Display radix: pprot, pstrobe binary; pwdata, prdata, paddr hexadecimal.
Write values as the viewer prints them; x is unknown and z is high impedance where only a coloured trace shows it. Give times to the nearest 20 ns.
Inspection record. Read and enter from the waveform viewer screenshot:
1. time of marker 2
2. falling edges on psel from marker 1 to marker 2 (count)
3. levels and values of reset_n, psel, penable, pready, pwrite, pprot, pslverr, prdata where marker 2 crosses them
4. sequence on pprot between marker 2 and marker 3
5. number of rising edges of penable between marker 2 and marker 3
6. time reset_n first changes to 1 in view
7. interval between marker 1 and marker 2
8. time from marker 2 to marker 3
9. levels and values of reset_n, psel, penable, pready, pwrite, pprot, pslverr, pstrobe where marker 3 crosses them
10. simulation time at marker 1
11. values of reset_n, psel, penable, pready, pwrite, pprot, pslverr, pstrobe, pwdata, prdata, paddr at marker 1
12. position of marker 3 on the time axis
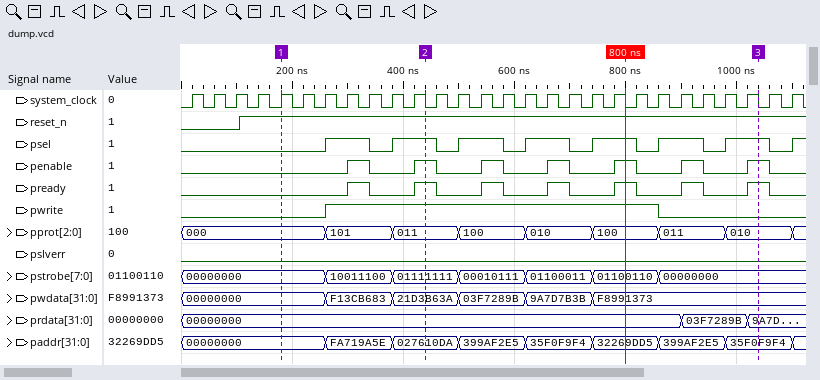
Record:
440 ns
1
reset_n=1, psel=1, penable=1, pready=1, pwrite=1, pprot=011, pslverr=0, prdata=00000000
011, 100, 010, 100, 011, 010
5
100 ns
260 ns
600 ns
reset_n=1, psel=1, penable=1, pready=1, pwrite=0, pprot=010, pslverr=0, pstrobe=00000000
180 ns
reset_n=1, psel=0, penable=0, pready=0, pwrite=0, pprot=000, pslverr=0, pstrobe=00000000, pwdata=00000000, prdata=00000000, paddr=00000000
1040 ns
